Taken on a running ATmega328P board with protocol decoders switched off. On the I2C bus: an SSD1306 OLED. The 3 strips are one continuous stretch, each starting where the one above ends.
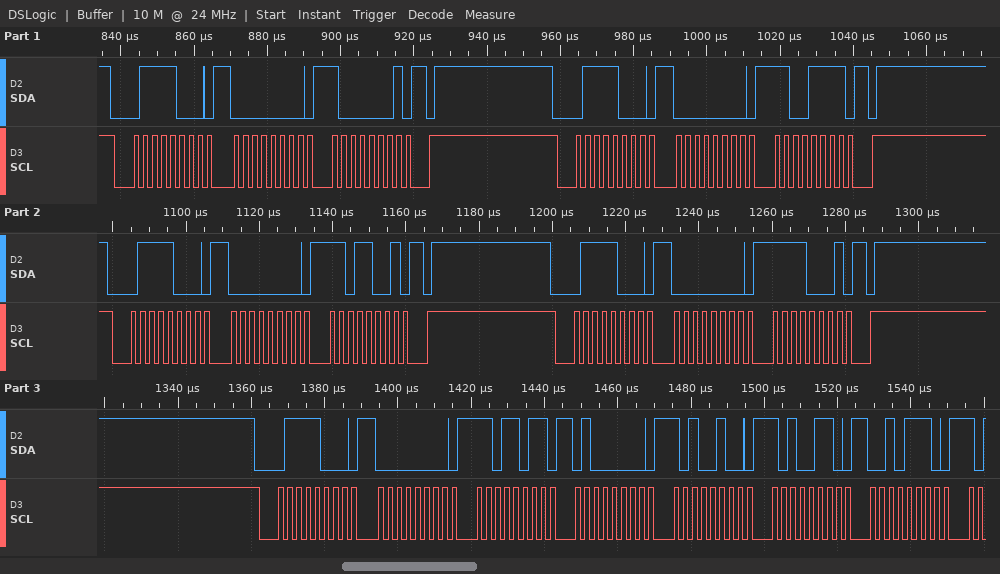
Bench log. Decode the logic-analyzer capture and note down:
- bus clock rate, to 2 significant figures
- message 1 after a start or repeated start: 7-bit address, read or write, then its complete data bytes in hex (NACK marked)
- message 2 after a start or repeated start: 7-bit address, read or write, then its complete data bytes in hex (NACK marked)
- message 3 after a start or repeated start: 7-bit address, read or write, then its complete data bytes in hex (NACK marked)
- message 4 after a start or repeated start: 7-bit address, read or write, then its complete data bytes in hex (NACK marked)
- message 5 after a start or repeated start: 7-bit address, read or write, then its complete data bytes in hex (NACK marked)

400 kHz
0x3C write: 00 81
0x3C write: 00 CF
0x3C write: 00 D9
0x3C write: 00 F1
0x3C write: 00 DB 40 A4 A6 2E
